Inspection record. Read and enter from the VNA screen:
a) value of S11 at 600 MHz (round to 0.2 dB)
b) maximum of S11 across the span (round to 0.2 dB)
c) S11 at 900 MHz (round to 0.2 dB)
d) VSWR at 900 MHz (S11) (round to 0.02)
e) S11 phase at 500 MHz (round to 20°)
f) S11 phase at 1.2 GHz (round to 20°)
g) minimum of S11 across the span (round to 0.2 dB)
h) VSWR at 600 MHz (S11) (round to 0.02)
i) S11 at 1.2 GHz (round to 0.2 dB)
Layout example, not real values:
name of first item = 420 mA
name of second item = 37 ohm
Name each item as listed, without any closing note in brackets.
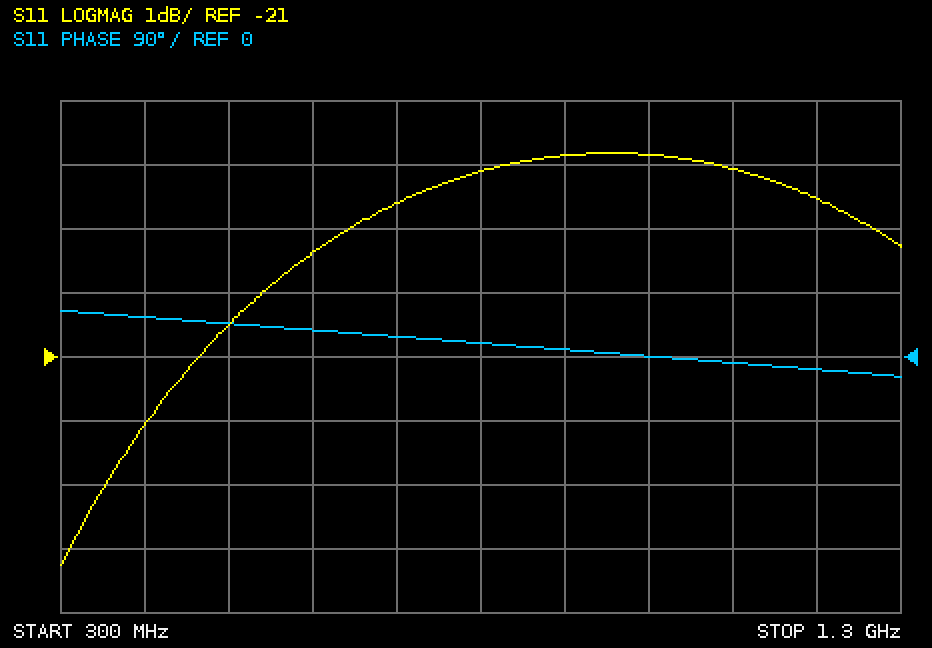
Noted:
value of S11 at 600 MHz = -19.4 dB
maximum of S11 across the span = -17.8 dB
S11 at 900 MHz = -17.8 dB
VSWR at 900 MHz (S11) = 1.30
S11 phase at 500 MHz = 40°
S11 phase at 1.2 GHz = -20°
minimum of S11 across the span = -24.2 dB
VSWR at 600 MHz (S11) = 1.24
S11 at 1.2 GHz = -18.6 dB
